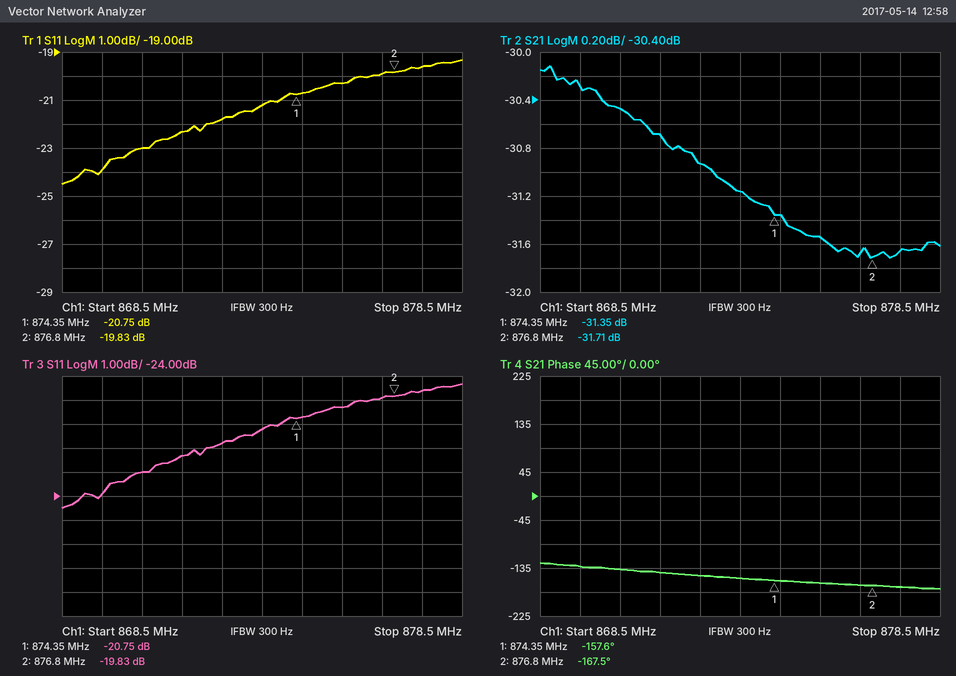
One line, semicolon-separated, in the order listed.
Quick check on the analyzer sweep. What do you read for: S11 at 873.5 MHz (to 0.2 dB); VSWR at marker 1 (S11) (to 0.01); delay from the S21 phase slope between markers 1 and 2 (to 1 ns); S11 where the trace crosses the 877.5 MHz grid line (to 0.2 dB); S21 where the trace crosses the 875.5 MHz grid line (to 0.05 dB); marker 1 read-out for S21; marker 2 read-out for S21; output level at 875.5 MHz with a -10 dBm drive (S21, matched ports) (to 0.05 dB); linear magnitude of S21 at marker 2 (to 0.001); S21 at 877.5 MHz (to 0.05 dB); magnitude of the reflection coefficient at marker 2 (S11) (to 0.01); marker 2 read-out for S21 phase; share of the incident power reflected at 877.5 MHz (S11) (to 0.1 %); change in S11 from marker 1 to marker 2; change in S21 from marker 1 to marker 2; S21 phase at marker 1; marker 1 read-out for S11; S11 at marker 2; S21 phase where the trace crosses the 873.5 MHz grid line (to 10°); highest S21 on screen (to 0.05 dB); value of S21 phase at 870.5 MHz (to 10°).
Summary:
-21.2 dB; 1.20; 11 ns; -19.6 dB; -31.55 dB; -31.35 dB; -31.71 dB; -41.55 dBm; 0.026; -31.65 dB; 0.10; -167.5°; 1.1 %; 0.92 dB; -0.36 dB; -157.6°; -20.75 dB; -19.83 dB; -150°; -30.10 dB; -140°
